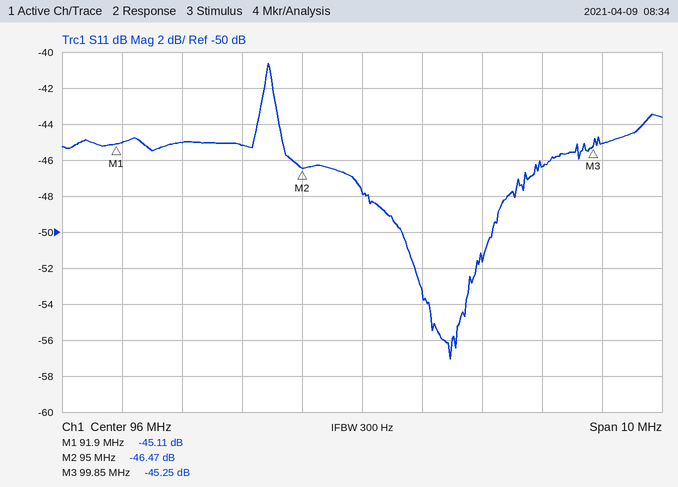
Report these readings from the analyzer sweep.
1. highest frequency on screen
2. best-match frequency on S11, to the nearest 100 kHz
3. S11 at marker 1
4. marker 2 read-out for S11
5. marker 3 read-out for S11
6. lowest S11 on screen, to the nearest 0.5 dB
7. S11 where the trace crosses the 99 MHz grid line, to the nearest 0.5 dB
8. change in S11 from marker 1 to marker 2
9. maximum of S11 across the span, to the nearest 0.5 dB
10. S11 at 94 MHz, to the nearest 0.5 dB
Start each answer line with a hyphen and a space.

- 101 MHz
- 97.5 MHz
- -45.11 dB
- -46.47 dB
- -45.25 dB
- -57.0 dB
- -46.5 dB
- -1.36 dB
- -40.5 dB
- -45.0 dB
